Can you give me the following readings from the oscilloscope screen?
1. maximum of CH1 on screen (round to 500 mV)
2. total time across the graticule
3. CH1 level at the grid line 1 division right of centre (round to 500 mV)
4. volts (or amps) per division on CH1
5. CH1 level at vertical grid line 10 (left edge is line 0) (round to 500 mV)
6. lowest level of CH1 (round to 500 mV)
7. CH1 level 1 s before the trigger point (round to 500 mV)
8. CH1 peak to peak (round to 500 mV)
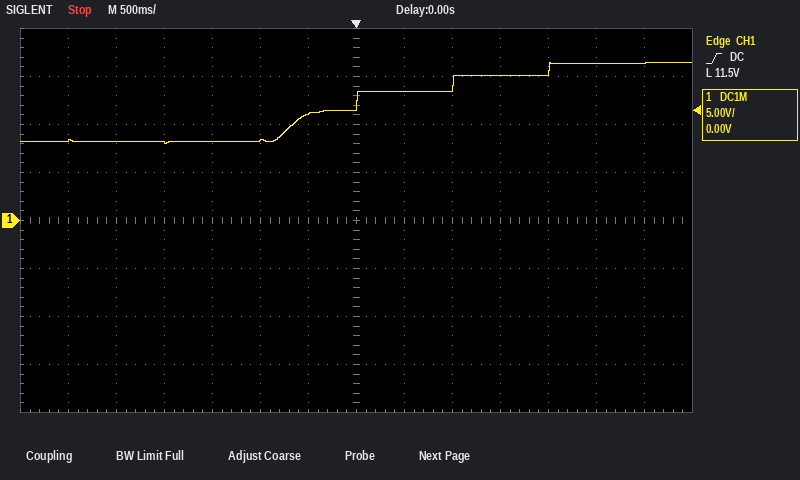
16.5 V
7 s
13.5 V
5 V
15.0 V
8.0 V
8.5 V
8.5 V
